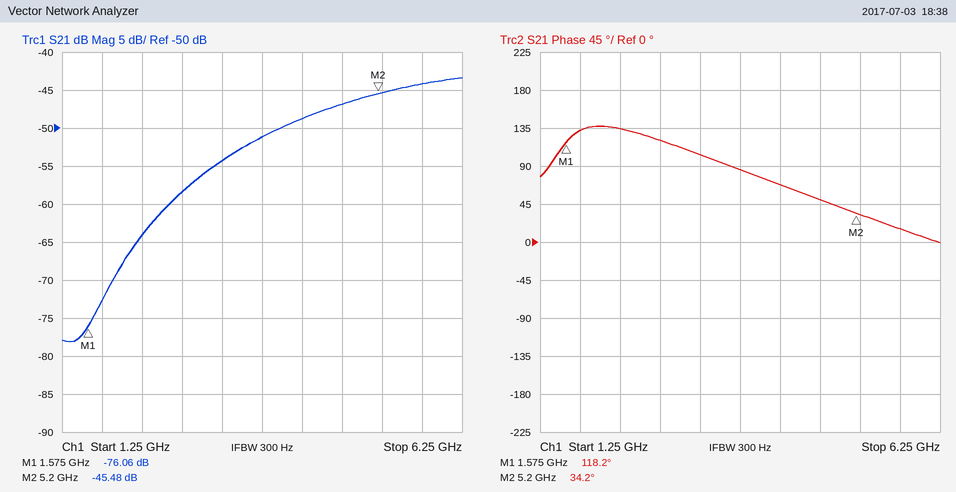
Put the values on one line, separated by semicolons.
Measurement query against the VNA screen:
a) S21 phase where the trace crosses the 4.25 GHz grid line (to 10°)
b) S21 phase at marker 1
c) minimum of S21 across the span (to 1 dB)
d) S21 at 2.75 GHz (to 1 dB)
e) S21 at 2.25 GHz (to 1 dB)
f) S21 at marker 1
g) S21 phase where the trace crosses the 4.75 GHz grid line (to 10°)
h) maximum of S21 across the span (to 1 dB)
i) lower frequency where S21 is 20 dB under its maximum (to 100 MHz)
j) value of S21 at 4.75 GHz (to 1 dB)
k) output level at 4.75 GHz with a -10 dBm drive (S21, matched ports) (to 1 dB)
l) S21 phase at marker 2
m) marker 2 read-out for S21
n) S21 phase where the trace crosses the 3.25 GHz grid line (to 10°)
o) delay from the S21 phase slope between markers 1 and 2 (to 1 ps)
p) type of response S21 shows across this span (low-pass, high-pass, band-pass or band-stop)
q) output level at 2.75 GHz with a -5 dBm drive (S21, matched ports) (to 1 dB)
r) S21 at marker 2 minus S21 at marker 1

70°; 118.2°; -78 dB; -58 dB; -64 dB; -76.06 dB; 50°; -43 dB; 2.3 GHz; -47 dB; -57 dBm; 34.2°; -45.48 dB; 100°; 64 ps; high-pass; -63 dBm; 30.58 dB
